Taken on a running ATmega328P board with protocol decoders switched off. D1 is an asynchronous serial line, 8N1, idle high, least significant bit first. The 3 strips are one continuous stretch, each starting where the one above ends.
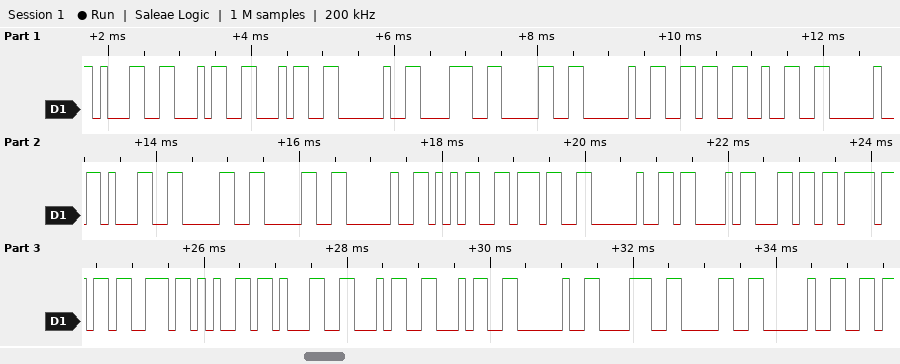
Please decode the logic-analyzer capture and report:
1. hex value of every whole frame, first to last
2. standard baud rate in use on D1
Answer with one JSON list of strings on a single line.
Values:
["31 34 34 20 38 30 20 36 32 20 31 30 30 20 35 37 20 43 6C 6F 73 65 31 34 34 20 38 30 20", "9600 baud"]
